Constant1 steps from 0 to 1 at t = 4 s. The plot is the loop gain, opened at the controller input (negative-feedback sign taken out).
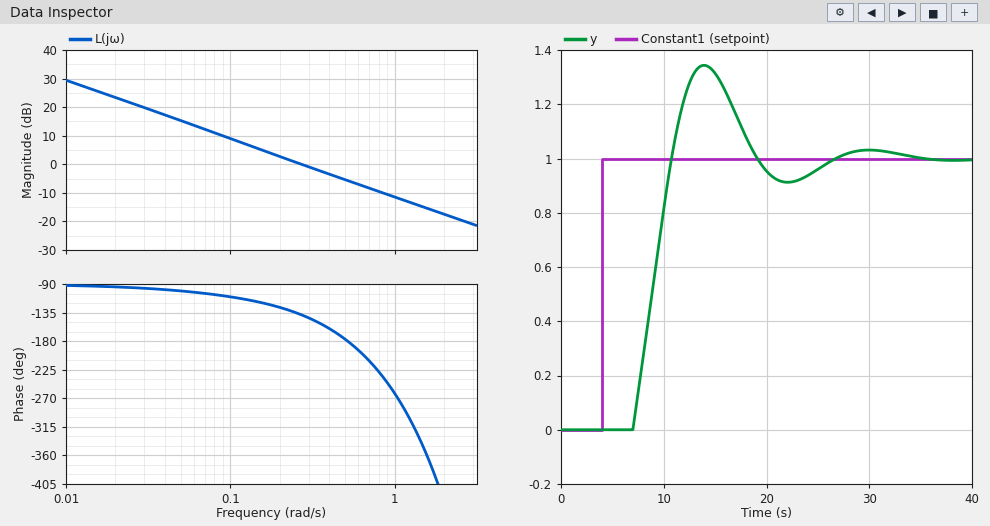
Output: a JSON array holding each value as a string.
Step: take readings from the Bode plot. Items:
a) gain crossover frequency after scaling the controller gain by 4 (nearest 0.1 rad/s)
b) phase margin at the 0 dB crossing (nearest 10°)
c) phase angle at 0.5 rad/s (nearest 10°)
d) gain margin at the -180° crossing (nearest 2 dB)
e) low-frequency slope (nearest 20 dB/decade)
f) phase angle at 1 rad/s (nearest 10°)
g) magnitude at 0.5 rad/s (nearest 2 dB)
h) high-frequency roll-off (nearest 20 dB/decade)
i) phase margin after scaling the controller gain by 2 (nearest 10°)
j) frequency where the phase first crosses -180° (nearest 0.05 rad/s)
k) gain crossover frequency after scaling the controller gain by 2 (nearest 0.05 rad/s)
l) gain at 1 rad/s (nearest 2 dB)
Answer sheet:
["1.1 rad/s", "40°", "-180°", "6 dB", "-20 dB/decade", "-260°", "-6 dB", "-20 dB/decade", "0°", "0.50 rad/s", "0.55 rad/s", "-12 dB"]
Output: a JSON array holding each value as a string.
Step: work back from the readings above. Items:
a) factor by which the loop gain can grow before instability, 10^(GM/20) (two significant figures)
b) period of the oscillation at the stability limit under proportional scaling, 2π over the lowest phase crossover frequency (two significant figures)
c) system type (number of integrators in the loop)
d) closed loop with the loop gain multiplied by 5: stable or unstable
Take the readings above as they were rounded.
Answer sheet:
["2.0", "13 s", "1", "unstable"]
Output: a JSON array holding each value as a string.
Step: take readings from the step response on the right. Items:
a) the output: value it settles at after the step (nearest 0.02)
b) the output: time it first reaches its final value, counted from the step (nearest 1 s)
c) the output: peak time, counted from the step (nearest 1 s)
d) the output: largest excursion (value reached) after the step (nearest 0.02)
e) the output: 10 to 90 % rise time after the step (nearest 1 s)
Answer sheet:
["1.00", "7 s", "10 s", "1.34", "3 s"]
